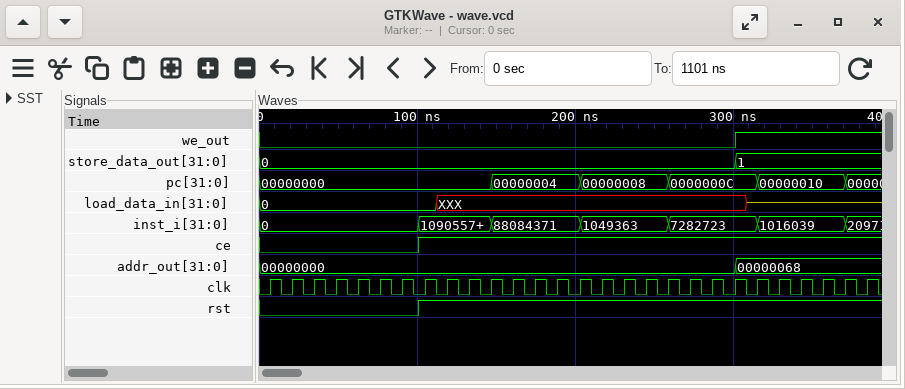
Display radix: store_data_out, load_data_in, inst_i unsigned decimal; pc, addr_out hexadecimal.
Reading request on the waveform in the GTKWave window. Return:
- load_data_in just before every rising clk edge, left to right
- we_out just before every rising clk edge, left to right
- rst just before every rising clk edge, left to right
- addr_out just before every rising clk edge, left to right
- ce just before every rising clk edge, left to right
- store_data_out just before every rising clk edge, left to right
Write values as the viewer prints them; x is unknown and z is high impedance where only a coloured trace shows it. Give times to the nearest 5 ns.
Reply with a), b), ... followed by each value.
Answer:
a) 0, 0, 0, 0, 0, 0, 0, 0, XXX, XXX, XXX, XXX, XXX, XXX, XXX, XXX, XXX, XXX, XXX, XXX, XXX, XXX, z, z, z, z, z, z
b) 0 0 0 0 0 0 0 0 0 0 0 0 0 0 0 0 0 0 0 0 0 0 1 1 1 1 1 1
c) 0 0 0 0 0 0 0 1 1 1 1 1 1 1 1 1 1 1 1 1 1 1 1 1 1 1 1 1
d) 00000000, 00000000, 00000000, 00000000, 00000000, 00000000, 00000000, 00000000, 00000000, 00000000, 00000000, 00000000, 00000000, 00000000, 00000000, 00000000, 00000000, 00000000, 00000000, 00000000, 00000000, 00000000, 00000068, 00000068, 00000068, 00000068, 00000068, 00000068
e) 0 0 0 0 0 0 0 1 1 1 1 1 1 1 1 1 1 1 1 1 1 1 1 1 1 1 1 1
f) 0, 0, 0, 0, 0, 0, 0, 0, 0, 0, 0, 0, 0, 0, 0, 0, 0, 0, 0, 0, 0, 0, 1, 1, 1, 1, 1, 1
